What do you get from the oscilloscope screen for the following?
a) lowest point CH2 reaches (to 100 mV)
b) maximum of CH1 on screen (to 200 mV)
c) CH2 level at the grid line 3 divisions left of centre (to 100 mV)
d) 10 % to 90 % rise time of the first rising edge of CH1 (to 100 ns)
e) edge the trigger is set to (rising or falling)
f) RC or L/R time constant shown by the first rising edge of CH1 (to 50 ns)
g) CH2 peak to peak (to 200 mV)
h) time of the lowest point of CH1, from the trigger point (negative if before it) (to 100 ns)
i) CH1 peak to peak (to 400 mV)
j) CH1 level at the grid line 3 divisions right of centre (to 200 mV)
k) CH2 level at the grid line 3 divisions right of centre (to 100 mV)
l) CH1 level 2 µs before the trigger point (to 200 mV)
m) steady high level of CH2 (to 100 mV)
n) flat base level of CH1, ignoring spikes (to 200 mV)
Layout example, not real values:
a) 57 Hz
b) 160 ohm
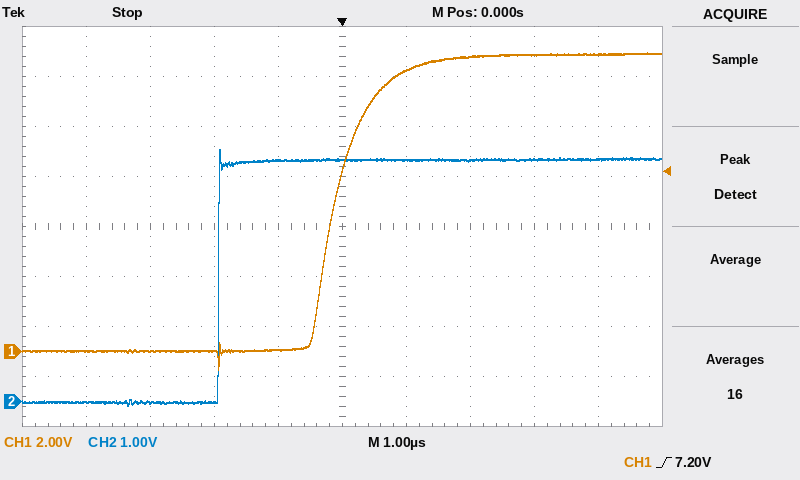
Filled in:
a) -100 mV
b) 12.0 V
c) 0.0 V
d) 1.1 µs
e) rising
f) 500 ns
g) 5.2 V
h) -1.9 µs
i) 12.8 V
j) 11.8 V
k) 4.8 V
l) 0.0 V
m) 4.8 V
n) 0.0 V
